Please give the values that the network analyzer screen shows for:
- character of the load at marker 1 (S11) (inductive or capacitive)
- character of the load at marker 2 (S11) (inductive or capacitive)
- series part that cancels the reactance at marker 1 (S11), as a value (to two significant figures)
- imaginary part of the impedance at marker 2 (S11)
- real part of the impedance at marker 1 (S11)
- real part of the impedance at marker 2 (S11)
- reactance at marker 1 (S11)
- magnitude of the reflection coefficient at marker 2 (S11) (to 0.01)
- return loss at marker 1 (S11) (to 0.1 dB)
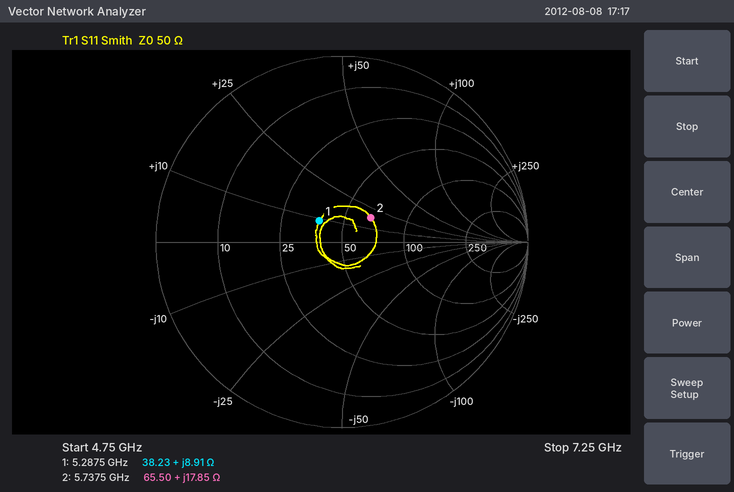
inductive
inductive
3.4 pF
+17.85 Ω
38.23 Ω
65.50 Ω
+8.91 Ω
0.20
15.6 dB
